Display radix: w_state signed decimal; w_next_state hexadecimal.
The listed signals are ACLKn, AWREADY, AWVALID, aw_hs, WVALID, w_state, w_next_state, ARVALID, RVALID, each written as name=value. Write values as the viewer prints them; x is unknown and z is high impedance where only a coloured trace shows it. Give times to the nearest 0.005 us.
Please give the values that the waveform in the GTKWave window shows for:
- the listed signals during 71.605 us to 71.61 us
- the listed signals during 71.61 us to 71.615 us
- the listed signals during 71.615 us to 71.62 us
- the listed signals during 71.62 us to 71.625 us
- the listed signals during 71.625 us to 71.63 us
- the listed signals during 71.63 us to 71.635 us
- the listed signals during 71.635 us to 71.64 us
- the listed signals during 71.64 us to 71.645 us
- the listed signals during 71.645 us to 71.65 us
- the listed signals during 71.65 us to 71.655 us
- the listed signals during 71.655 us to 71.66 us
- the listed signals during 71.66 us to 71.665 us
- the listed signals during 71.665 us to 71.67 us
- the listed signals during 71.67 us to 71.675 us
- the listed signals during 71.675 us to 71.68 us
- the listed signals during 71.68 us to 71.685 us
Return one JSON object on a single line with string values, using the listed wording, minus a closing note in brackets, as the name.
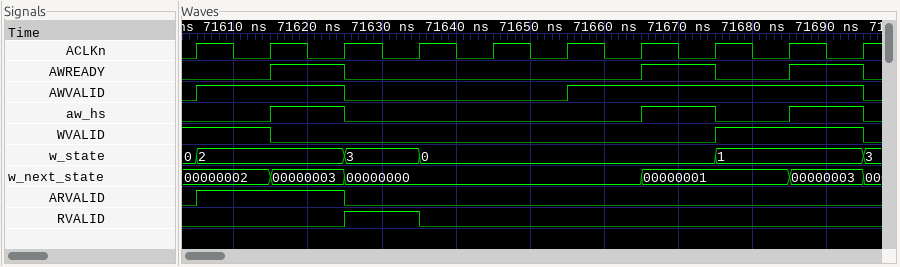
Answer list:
{"the listed signals during 71.605 us to 71.61 us": "ACLKn=1, AWREADY=0, AWVALID=1, aw_hs=0, WVALID=1, w_state=2, w_next_state=00000002, ARVALID=1, RVALID=0", "the listed signals during 71.61 us to 71.615 us": "ACLKn=0, AWREADY=0, AWVALID=1, aw_hs=0, WVALID=1, w_state=2, w_next_state=00000002, ARVALID=1, RVALID=0", "the listed signals during 71.615 us to 71.62 us": "ACLKn=1, AWREADY=1, AWVALID=1, aw_hs=1, WVALID=0, w_state=2, w_next_state=00000003, ARVALID=1, RVALID=0", "the listed signals during 71.62 us to 71.625 us": "ACLKn=0, AWREADY=1, AWVALID=1, aw_hs=1, WVALID=0, w_state=2, w_next_state=00000003, ARVALID=1, RVALID=0", "the listed signals during 71.625 us to 71.63 us": "ACLKn=1, AWREADY=0, AWVALID=0, aw_hs=0, WVALID=0, w_state=3, w_next_state=00000000, ARVALID=0, RVALID=1", "the listed signals during 71.63 us to 71.635 us": "ACLKn=0, AWREADY=0, AWVALID=0, aw_hs=0, WVALID=0, w_state=3, w_next_state=00000000, ARVALID=0, RVALID=1", "the listed signals during 71.635 us to 71.64 us": "ACLKn=1, AWREADY=0, AWVALID=0, aw_hs=0, WVALID=0, w_state=0, w_next_state=00000000, ARVALID=0, RVALID=0", "the listed signals during 71.64 us to 71.645 us": "ACLKn=0, AWREADY=0, AWVALID=0, aw_hs=0, WVALID=0, w_state=0, w_next_state=00000000, ARVALID=0, RVALID=0", "the listed signals during 71.645 us to 71.65 us": "ACLKn=1, AWREADY=0, AWVALID=0, aw_hs=0, WVALID=0, w_state=0, w_next_state=00000000, ARVALID=0, RVALID=0", "the listed signals during 71.65 us to 71.655 us": "ACLKn=0, AWREADY=0, AWVALID=0, aw_hs=0, WVALID=0, w_state=0, w_next_state=00000000, ARVALID=0, RVALID=0", "the listed signals during 71.655 us to 71.66 us": "ACLKn=1, AWREADY=0, AWVALID=1, aw_hs=0, WVALID=0, w_state=0, w_next_state=00000000, ARVALID=0, RVALID=0", "the listed signals during 71.66 us to 71.665 us": "ACLKn=0, AWREADY=0, AWVALID=1, aw_hs=0, WVALID=0, w_state=0, w_next_state=00000000, ARVALID=0, RVALID=0", "the listed signals during 71.665 us to 71.67 us": "ACLKn=1, AWREADY=1, AWVALID=1, aw_hs=1, WVALID=0, w_state=0, w_next_state=00000001, ARVALID=0, RVALID=0", "the listed signals during 71.67 us to 71.675 us": "ACLKn=0, AWREADY=1, AWVALID=1, aw_hs=1, WVALID=0, w_state=0, w_next_state=00000001, ARVALID=0, RVALID=0", "the listed signals during 71.675 us to 71.68 us": "ACLKn=1, AWREADY=0, AWVALID=1, aw_hs=0, WVALID=1, w_state=1, w_next_state=00000001, ARVALID=0, RVALID=0", "the listed signals during 71.68 us to 71.685 us": "ACLKn=0, AWREADY=0, AWVALID=1, aw_hs=0, WVALID=1, w_state=1, w_next_state=00000001, ARVALID=0, RVALID=0"}
